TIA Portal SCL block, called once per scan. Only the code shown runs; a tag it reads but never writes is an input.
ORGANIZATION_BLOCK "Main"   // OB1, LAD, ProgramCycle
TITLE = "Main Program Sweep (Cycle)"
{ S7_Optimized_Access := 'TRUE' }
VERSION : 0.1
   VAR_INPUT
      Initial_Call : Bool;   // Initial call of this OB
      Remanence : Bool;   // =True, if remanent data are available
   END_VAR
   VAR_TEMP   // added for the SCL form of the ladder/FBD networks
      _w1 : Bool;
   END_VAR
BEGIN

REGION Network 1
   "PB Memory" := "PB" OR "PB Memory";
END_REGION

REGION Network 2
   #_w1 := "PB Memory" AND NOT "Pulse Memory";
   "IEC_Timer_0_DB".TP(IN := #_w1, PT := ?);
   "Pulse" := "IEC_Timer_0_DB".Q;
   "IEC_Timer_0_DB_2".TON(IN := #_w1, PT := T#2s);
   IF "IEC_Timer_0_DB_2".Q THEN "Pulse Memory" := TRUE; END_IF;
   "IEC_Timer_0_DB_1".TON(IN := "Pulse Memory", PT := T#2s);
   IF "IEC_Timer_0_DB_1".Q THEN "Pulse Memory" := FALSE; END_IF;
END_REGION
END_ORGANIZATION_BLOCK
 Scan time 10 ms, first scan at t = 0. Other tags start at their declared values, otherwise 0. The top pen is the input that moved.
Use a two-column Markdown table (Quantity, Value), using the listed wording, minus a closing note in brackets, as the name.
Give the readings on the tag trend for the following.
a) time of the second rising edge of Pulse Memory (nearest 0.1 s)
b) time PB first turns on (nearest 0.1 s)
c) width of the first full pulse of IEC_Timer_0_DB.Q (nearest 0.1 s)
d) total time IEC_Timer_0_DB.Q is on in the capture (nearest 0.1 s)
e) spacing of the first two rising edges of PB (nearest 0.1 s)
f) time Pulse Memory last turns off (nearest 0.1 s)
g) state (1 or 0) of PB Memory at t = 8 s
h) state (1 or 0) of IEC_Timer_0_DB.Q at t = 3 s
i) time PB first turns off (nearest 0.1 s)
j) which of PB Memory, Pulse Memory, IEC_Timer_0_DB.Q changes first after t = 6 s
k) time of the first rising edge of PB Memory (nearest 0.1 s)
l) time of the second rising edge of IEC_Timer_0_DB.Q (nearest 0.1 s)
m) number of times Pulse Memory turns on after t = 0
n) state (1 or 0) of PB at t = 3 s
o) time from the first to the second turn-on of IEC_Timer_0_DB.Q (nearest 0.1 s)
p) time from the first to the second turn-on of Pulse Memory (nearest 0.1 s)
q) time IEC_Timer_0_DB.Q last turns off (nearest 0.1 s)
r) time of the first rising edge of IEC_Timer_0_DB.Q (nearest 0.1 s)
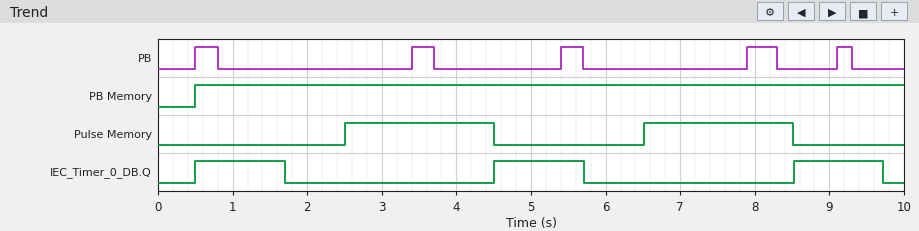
| Quantity | Value |
|---|---|
| time of the second rising edge of Pulse Memory | 6.5 s |
| time PB first turns on | 0.5 s |
| width of the first full pulse of IEC_Timer_0_DB.Q | 1.2 s |
| total time IEC_Timer_0_DB.Q is on in the capture | 3.6 s |
| spacing of the first two rising edges of PB | 2.9 s |
| time Pulse Memory last turns off | 8.5 s |
| state (1 or 0) of PB Memory at t = 8 s | 1 |
| state (1 or 0) of IEC_Timer_0_DB.Q at t = 3 s | 0 |
| time PB first turns off | 0.8 s |
| which of PB Memory, Pulse Memory, IEC_Timer_0_DB.Q changes first after t = 6 s | Pulse Memory |
| time of the first rising edge of PB Memory | 0.5 s |
| time of the second rising edge of IEC_Timer_0_DB.Q | 4.5 s |
| number of times Pulse Memory turns on after t = 0 | 2 |
| state (1 or 0) of PB at t = 3 s | 0 |
| time from the first to the second turn-on of IEC_Timer_0_DB.Q | 4.0 s |
| time from the first to the second turn-on of Pulse Memory | 4.0 s |
| time IEC_Timer_0_DB.Q last turns off | 9.7 s |
| time of the first rising edge of IEC_Timer_0_DB.Q | 0.5 s |
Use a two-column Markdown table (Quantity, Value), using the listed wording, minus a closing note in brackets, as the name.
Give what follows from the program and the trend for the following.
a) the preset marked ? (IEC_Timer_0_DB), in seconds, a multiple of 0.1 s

| Quantity | Value |
|---|---|
| the preset marked ? (IEC_Timer_0_DB), in seconds, a multiple of 0.1 s | 1.2 s |
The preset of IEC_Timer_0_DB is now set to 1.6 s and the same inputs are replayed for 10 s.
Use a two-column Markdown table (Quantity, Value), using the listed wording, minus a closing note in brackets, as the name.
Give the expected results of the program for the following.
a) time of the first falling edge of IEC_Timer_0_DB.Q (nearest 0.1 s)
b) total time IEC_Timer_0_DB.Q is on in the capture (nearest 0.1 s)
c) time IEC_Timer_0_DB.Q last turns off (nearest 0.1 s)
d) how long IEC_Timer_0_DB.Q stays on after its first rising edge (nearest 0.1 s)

| Quantity | Value |
|---|---|
| time of the first falling edge of IEC_Timer_0_DB.Q | 2.1 s |
| total time IEC_Timer_0_DB.Q is on in the capture | 4.7 s |
| time IEC_Timer_0_DB.Q last turns off | 6.1 s |
| how long IEC_Timer_0_DB.Q stays on after its first rising edge | 1.6 s |
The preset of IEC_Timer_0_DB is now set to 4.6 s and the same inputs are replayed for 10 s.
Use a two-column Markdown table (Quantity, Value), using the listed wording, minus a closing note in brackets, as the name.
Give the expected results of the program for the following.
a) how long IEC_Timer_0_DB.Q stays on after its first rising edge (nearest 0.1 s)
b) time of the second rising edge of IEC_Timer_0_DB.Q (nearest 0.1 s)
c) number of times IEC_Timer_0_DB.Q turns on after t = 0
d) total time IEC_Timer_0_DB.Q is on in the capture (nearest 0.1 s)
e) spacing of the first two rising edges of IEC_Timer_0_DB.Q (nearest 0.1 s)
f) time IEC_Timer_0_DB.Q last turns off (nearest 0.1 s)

| Quantity | Value |
|---|---|
| how long IEC_Timer_0_DB.Q stays on after its first rising edge | 4.6 s |
| time of the second rising edge of IEC_Timer_0_DB.Q | 8.5 s |
| number of times IEC_Timer_0_DB.Q turns on after t = 0 | 2 |
| total time IEC_Timer_0_DB.Q is on in the capture | 6.1 s |
| spacing of the first two rising edges of IEC_Timer_0_DB.Q | 8.0 s |
| time IEC_Timer_0_DB.Q last turns off | 5.1 s |
